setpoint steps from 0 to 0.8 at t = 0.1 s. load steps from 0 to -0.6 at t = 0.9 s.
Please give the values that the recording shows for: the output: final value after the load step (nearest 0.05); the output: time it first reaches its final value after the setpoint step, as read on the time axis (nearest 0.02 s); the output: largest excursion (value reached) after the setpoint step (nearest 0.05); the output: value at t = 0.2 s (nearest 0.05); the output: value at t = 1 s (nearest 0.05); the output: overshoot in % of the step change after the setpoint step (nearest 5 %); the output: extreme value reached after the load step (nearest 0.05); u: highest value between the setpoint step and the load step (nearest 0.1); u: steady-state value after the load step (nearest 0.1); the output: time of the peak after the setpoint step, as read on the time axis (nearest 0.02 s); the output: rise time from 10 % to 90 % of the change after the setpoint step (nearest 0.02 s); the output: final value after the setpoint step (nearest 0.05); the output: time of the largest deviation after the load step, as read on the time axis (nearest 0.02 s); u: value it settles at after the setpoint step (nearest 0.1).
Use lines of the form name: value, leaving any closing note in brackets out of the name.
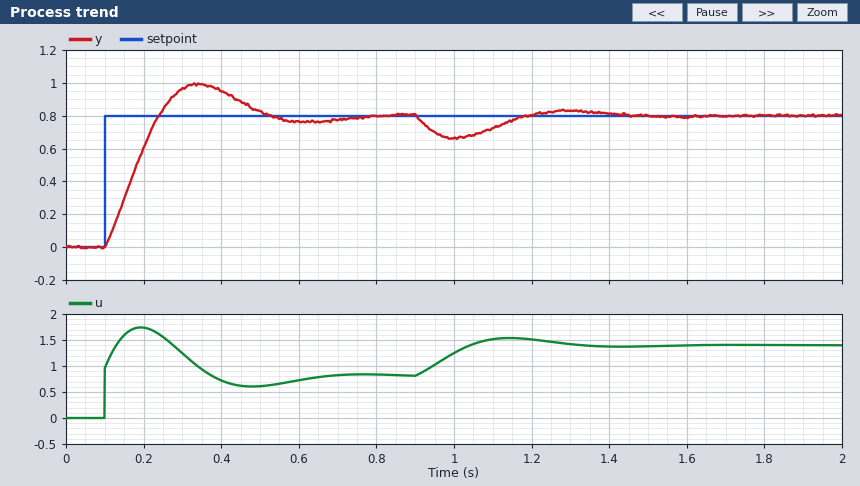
the output: final value after the load step: 0.80
the output: time it first reaches its final value after the setpoint step, as read on the time axis: 0.24 s
the output: largest excursion (value reached) after the setpoint step: 1.00
the output: value at t = 0.2 s: 0.60
the output: value at t = 1 s: 0.65
the output: overshoot in % of the step change after the setpoint step: 25 %
the output: extreme value reached after the load step: 0.65
u: highest value between the setpoint step and the load step: 1.7
u: steady-state value after the load step: 1.4
the output: time of the peak after the setpoint step, as read on the time axis: 0.34 s
the output: rise time from 10 % to 90 % of the change after the setpoint step: 0.10 s
the output: final value after the setpoint step: 0.80
the output: time of the largest deviation after the load step, as read on the time axis: 1.00 s
u: value it settles at after the setpoint step: 0.8
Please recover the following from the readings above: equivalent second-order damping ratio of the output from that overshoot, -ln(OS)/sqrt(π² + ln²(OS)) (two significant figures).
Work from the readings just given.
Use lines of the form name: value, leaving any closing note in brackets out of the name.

equivalent second-order damping ratio of the output from that overshoot, -ln(OS)/sqrt(π² + ln²(OS)): 0.40
